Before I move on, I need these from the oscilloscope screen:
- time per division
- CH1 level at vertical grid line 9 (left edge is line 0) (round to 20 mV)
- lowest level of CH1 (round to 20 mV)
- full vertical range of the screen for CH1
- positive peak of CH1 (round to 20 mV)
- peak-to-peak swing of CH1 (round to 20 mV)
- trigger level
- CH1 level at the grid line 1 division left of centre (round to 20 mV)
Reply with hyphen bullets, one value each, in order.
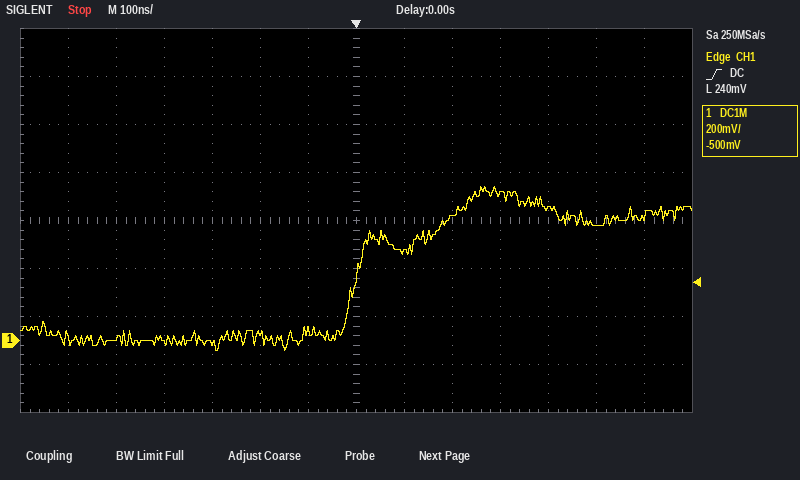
- 100 ns
- 520 mV
- -40 mV
- 1.6 V
- 640 mV
- 680 mV
- 240 mV
- 40 mV
